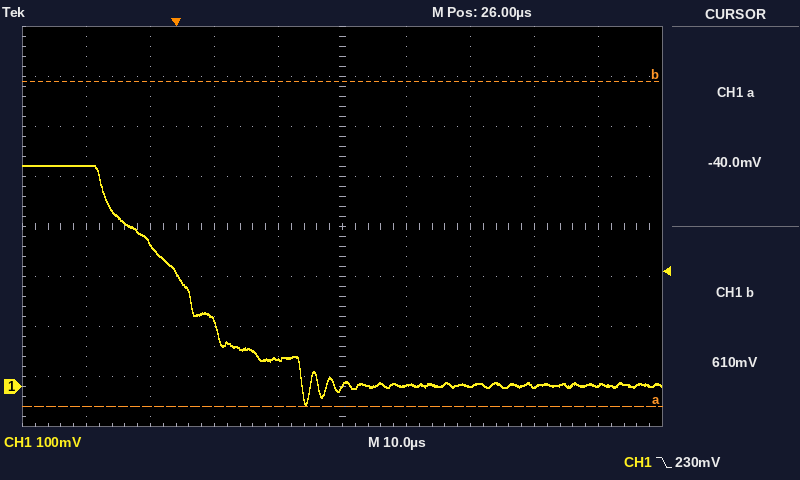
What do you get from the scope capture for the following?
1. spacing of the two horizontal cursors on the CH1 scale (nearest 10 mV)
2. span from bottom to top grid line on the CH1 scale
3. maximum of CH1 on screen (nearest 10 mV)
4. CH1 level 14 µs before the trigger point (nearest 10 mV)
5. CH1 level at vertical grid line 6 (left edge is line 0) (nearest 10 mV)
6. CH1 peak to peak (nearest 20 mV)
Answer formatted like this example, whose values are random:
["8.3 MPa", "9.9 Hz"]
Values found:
["650 mV", "800 mV", "440 mV", "440 mV", "0 mV", "480 mV"]
